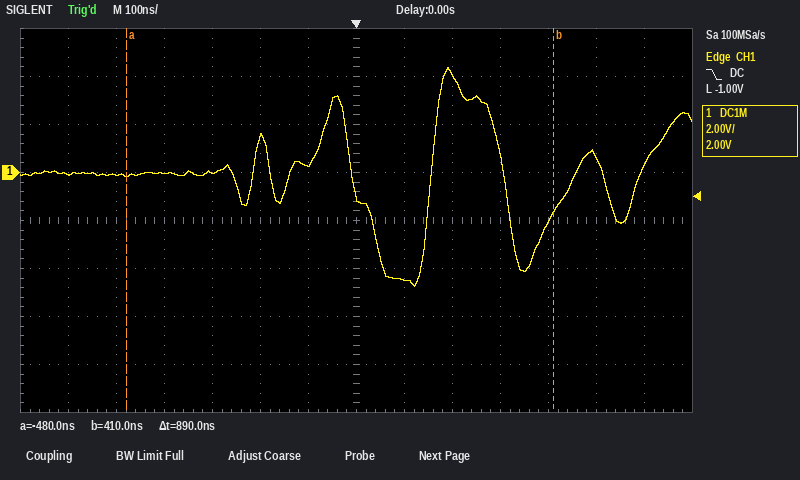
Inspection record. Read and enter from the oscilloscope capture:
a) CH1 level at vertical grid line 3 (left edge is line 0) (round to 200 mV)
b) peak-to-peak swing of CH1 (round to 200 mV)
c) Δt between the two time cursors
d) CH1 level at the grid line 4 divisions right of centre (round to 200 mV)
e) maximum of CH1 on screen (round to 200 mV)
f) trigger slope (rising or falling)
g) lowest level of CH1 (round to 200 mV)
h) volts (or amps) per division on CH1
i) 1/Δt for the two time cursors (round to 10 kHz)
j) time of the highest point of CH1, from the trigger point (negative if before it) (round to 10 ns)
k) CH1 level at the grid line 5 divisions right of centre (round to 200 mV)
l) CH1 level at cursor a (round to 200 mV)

0.0 V
9.2 V
890 ns
-2.0 V
4.4 V
falling
-4.8 V
2 V
1.12 MHz
+190 ns
600 mV
-200 mV
